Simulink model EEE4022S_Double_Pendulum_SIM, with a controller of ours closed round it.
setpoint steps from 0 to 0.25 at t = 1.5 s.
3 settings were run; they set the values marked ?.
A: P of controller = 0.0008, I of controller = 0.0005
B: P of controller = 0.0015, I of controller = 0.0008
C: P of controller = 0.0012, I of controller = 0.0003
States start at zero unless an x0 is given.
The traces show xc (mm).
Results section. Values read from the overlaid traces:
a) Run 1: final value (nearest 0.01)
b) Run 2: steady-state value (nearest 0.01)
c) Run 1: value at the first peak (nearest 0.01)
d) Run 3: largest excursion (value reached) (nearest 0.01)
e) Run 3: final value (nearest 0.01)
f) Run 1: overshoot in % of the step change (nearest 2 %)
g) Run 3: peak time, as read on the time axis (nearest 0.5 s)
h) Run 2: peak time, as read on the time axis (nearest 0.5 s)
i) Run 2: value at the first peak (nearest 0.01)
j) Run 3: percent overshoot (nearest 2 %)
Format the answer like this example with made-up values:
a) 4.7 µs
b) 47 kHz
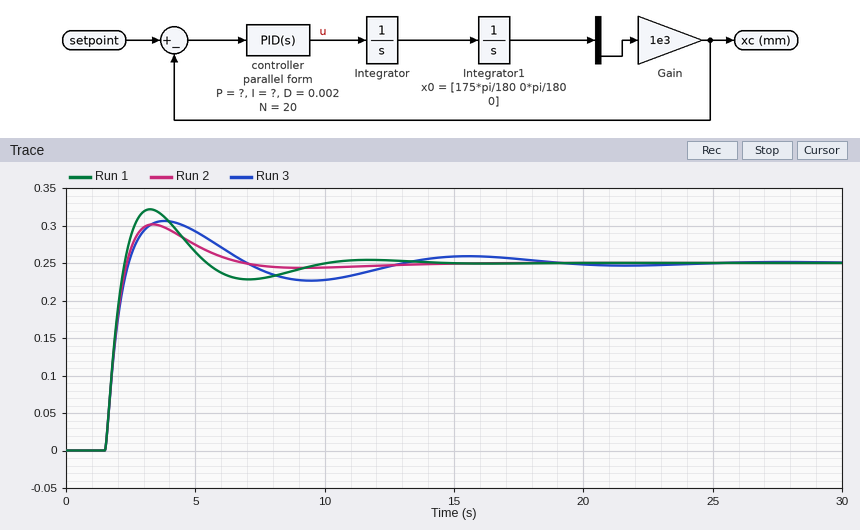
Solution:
a) 0.25
b) 0.25
c) 0.32
d) 0.31
e) 0.25
f) 28 %
g) 4.0 s
h) 3.5 s
i) 0.30
j) 22 %
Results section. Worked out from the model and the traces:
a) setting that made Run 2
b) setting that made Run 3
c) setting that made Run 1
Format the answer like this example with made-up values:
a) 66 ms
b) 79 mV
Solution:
a) C
b) A
c) B
